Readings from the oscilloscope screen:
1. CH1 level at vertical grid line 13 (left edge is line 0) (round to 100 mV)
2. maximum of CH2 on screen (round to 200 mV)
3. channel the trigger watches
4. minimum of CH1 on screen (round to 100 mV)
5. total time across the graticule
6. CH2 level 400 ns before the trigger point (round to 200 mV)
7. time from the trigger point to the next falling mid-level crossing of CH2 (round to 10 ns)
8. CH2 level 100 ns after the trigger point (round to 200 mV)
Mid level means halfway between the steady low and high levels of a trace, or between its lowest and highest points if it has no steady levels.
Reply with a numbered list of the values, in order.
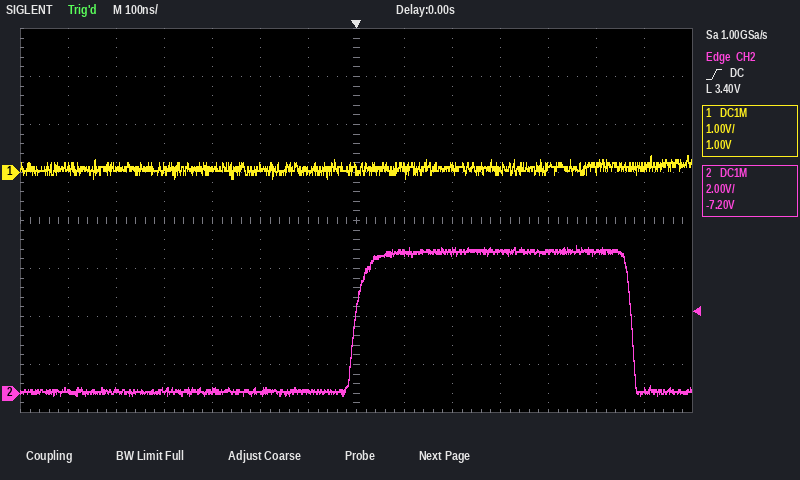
1. 100 mV
2. 6.2 V
3. CH2
4. -100 mV
5. 1.4 µs
6. 200 mV
7. 570 ns
8. 5.8 V
